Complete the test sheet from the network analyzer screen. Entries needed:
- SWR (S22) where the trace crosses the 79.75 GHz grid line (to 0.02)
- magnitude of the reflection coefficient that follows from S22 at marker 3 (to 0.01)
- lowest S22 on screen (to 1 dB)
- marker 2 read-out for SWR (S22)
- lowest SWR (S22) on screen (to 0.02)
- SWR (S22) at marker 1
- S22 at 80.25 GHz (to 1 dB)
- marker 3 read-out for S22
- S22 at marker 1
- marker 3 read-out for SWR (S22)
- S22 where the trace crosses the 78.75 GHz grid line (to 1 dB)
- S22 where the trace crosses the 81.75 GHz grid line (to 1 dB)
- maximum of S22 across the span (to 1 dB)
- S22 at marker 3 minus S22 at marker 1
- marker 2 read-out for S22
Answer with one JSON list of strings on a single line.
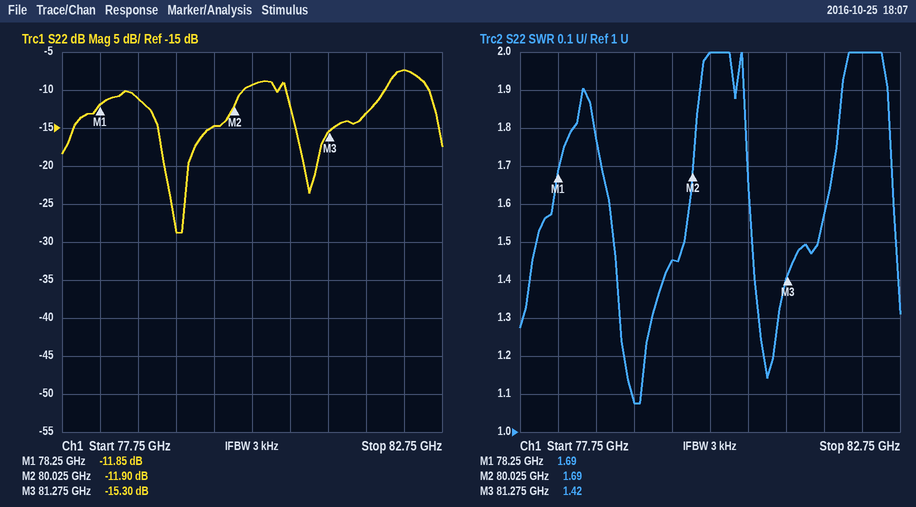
["1.46", "0.17", "-29 dB", "1.69", "1.08", "1.69", "-9 dB", "-15.30 dB", "-11.85 dB", "1.42", "-11 dB", "-13 dB", "-7 dB", "-3.45 dB", "-11.90 dB"]
